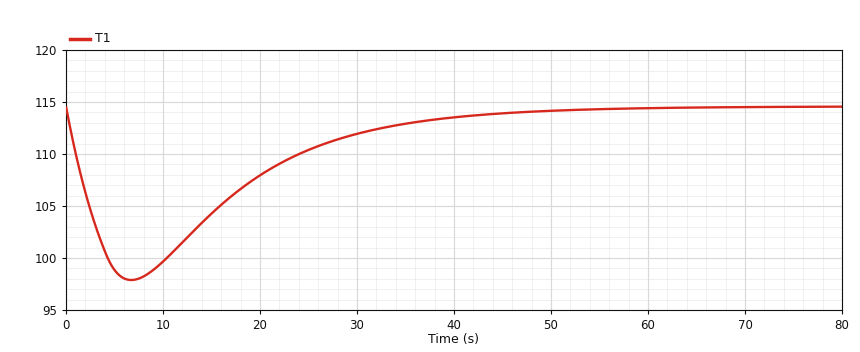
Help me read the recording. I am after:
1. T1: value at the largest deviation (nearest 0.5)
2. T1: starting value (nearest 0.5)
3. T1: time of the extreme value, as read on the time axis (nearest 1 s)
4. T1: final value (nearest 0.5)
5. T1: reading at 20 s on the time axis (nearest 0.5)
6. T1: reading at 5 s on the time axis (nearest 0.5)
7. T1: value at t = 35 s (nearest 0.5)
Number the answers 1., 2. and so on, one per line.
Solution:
1. 98.0
2. 114.5
3. 7 s
4. 114.5
5. 108.0
6. 99.0
7. 113.0
